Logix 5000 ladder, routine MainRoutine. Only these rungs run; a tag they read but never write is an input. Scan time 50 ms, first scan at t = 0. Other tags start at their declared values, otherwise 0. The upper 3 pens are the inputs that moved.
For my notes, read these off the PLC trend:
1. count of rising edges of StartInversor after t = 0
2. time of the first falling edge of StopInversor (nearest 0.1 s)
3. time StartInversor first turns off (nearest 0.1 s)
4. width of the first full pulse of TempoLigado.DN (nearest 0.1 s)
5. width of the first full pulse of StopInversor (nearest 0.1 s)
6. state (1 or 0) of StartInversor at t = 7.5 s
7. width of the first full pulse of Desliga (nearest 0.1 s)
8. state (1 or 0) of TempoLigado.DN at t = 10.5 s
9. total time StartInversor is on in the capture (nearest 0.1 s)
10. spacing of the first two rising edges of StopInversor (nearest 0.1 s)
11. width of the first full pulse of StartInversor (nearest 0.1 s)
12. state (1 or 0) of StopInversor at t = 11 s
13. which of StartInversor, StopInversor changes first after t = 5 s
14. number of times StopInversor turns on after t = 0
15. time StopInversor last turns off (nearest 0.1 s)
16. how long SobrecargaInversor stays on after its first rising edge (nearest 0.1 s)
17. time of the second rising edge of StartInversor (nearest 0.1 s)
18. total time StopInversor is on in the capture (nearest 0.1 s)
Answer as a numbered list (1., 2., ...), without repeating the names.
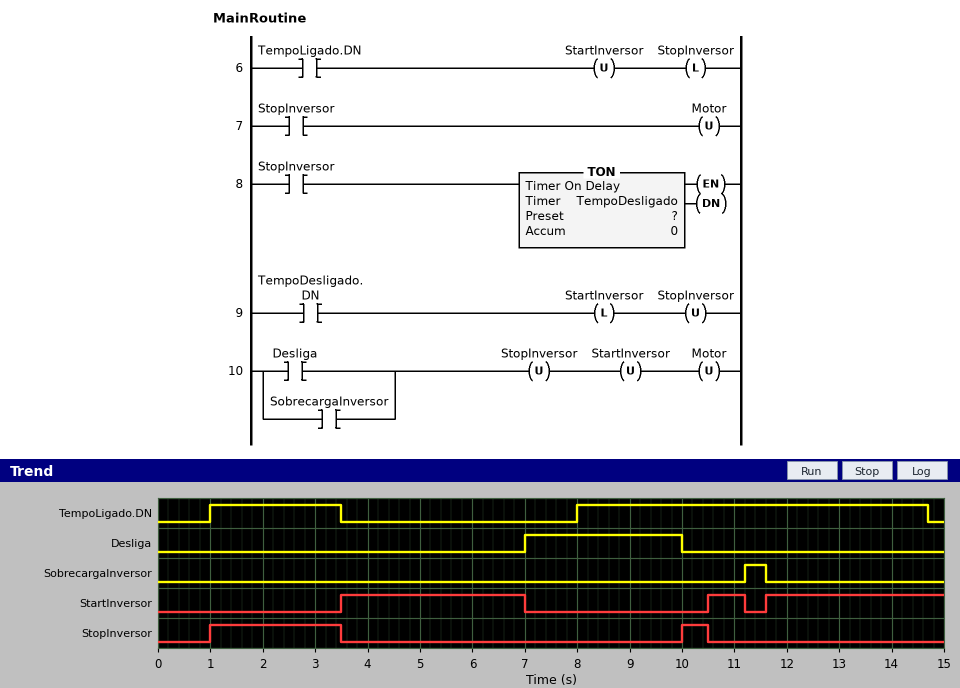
1. 3
2. 3.5 s
3. 7.0 s
4. 2.5 s
5. 2.5 s
6. 0
7. 3.0 s
8. 1
9. 7.6 s
10. 9.0 s
11. 3.5 s
12. 0
13. StartInversor
14. 2
15. 10.5 s
16. 0.4 s
17. 10.5 s
18. 3.0 s
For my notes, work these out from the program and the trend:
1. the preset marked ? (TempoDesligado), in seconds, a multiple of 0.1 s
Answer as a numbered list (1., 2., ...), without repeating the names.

1. 2.5 s
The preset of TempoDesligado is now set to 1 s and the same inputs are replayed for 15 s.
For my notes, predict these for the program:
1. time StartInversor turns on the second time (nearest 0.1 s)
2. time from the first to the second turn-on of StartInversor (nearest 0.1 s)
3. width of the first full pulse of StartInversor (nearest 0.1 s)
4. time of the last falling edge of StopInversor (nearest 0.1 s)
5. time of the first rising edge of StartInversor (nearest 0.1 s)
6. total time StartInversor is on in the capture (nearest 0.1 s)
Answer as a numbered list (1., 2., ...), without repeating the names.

1. 10.0 s
2. 8.0 s
3. 5.0 s
4. 2.0 s
5. 2.0 s
6. 9.6 s
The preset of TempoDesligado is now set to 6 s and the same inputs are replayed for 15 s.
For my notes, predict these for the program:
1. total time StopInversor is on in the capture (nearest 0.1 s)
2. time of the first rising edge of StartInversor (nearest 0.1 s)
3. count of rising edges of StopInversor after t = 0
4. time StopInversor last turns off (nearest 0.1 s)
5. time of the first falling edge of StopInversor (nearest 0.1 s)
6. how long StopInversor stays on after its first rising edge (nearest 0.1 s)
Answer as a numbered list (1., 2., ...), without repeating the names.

1. 9.6 s
2. 14.0 s
3. 3
4. 14.0 s
5. 7.0 s
6. 6.0 s
